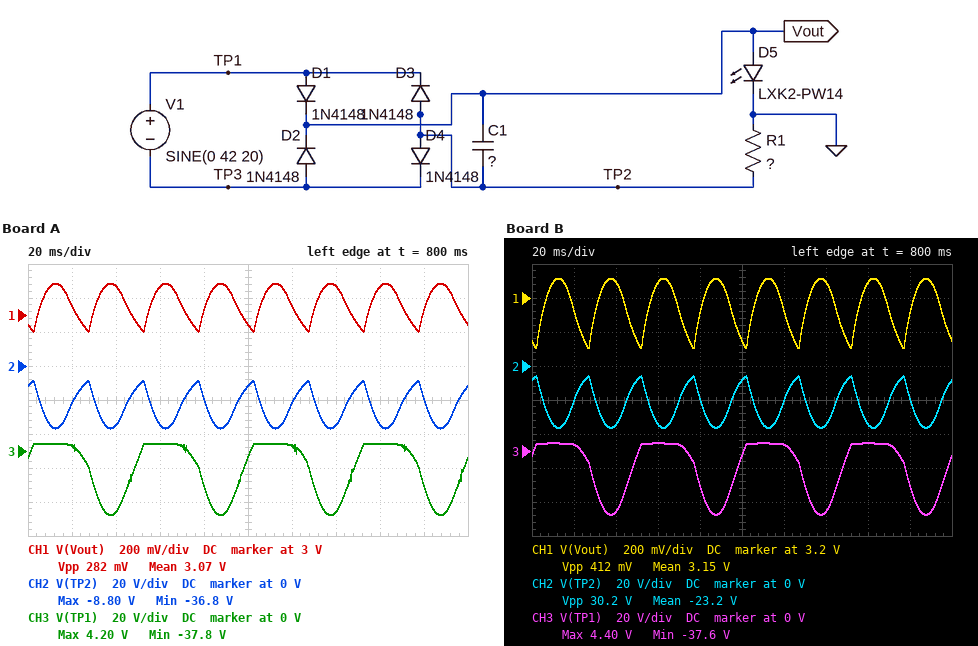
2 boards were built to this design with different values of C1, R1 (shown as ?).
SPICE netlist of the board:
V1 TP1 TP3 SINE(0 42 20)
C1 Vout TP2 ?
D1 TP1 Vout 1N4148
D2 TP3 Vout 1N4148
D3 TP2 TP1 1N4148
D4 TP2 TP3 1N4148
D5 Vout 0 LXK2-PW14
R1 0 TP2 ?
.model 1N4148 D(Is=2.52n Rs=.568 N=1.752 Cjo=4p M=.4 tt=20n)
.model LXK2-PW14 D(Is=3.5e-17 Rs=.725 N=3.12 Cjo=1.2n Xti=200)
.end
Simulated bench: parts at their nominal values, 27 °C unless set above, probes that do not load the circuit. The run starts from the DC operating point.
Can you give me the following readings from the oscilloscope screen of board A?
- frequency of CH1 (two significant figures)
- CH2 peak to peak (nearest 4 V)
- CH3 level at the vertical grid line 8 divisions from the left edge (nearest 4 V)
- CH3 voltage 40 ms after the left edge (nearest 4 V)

40 Hz
28 V
4 V
-36 V
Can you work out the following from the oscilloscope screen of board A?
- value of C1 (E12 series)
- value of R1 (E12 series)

68 µF
120 Ω
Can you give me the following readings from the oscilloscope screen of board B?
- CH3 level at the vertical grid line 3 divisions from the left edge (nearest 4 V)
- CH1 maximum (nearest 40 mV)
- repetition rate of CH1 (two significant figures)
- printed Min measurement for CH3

4 V
3.32 V
40 Hz
-37.6 V
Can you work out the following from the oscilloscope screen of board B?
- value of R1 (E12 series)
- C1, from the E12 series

82 Ω
68 µF
